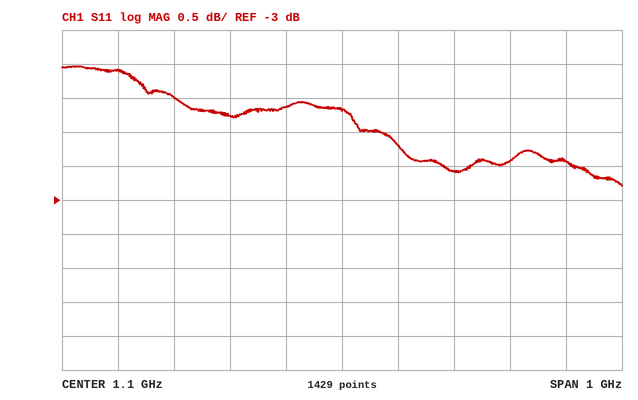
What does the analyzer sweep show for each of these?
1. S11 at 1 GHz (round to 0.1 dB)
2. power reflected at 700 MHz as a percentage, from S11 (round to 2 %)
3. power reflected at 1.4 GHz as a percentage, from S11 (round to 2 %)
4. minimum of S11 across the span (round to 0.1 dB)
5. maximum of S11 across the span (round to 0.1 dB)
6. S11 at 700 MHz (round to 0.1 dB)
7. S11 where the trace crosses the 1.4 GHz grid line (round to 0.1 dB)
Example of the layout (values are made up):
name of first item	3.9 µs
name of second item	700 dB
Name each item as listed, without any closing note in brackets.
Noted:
S11 at 1 GHz	-1.6 dB
power reflected at 700 MHz as a percentage, from S11	78 %
power reflected at 1.4 GHz as a percentage, from S11	58 %
minimum of S11 across the span	-2.8 dB
maximum of S11 across the span	-1.0 dB
S11 at 700 MHz	-1.1 dB
S11 where the trace crosses the 1.4 GHz grid line	-2.4 dB
